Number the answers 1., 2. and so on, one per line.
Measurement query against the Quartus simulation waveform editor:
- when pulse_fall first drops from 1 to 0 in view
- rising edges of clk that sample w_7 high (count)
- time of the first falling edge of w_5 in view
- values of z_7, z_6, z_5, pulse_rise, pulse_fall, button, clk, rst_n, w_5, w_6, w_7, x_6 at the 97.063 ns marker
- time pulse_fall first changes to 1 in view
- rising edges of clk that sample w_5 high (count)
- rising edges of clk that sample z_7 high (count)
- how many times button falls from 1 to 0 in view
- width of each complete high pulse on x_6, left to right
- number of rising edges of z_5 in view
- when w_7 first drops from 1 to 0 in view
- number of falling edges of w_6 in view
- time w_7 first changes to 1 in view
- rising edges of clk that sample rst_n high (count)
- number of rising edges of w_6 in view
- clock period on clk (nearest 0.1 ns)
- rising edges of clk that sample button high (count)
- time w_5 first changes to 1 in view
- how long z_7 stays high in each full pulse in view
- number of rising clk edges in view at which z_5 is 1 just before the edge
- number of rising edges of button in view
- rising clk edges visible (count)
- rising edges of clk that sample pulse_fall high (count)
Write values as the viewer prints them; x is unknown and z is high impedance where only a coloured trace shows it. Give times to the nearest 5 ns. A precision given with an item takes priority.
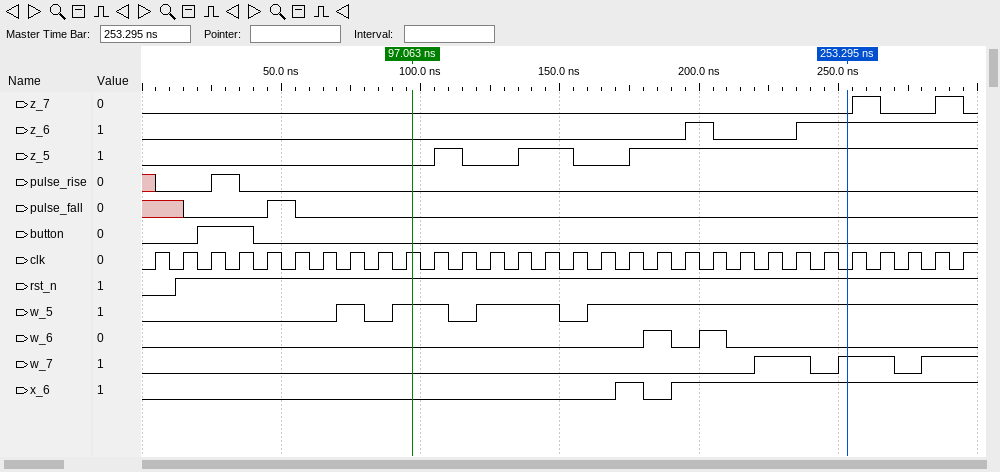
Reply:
1. 55 ns
2. 6
3. 80 ns
4. z_7=0, z_6=0, z_5=0, pulse_rise=0, pulse_fall=0, button=0, clk=1, rst_n=1, w_5=1, w_6=0, w_7=0, x_6=0
5. 45 ns
6. 20
7. 2
8. 1
9. 10 ns
10. 3
11. 240 ns
12. 2
13. 220 ns
14. 29
15. 2
16. 10 ns
17. 2
18. 70 ns
19. 10 ns, 10 ns
20. 15
21. 1
22. 30
23. 1
